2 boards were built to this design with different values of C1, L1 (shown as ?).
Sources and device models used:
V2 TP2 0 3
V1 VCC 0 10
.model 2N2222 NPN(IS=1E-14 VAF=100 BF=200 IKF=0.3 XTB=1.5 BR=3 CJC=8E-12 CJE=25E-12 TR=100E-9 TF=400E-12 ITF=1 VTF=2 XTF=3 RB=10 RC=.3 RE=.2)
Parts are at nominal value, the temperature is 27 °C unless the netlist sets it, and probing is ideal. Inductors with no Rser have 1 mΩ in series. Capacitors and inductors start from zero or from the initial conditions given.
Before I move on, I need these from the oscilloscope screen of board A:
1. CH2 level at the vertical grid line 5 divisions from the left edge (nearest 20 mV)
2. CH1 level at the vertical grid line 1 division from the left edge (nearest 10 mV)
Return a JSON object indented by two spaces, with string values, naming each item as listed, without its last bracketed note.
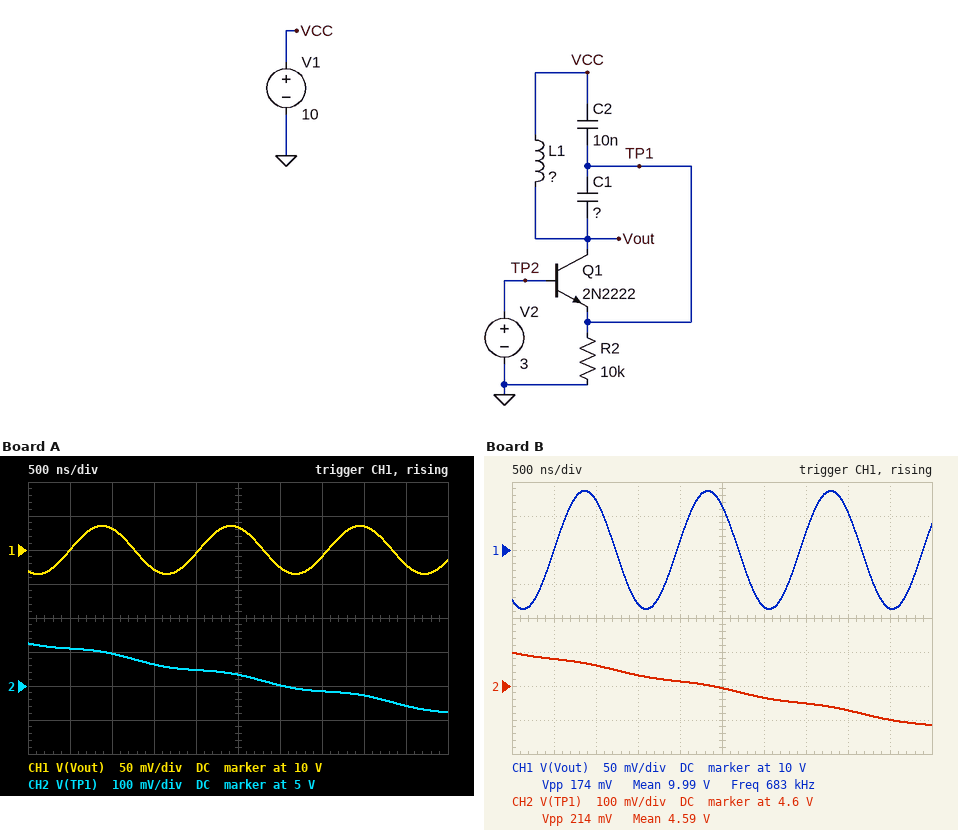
{
  "CH2 level at the vertical grid line 5 divisions from the left edge": "5.04 V",
  "CH1 level at the vertical grid line 1 division from the left edge": "10.00 V"
}
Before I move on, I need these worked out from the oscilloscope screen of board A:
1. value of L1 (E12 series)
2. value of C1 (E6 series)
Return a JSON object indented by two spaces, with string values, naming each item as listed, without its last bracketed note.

{
  "value of L1": "33 µH",
  "value of C1": "2.2 nF"
}
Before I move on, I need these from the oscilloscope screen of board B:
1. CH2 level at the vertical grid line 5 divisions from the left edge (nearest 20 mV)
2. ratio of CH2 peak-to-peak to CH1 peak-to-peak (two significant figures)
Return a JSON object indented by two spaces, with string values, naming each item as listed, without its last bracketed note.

{
  "CH2 level at the vertical grid line 5 divisions from the left edge": "4.60 V",
  "ratio of CH2 peak-to-peak to CH1 peak-to-peak": "1.2"
}
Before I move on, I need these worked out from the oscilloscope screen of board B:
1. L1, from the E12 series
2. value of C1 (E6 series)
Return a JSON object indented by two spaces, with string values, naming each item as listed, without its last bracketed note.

{
  "L1, from the E12 series": "120 µH",
  "value of C1": "470 pF"
}
